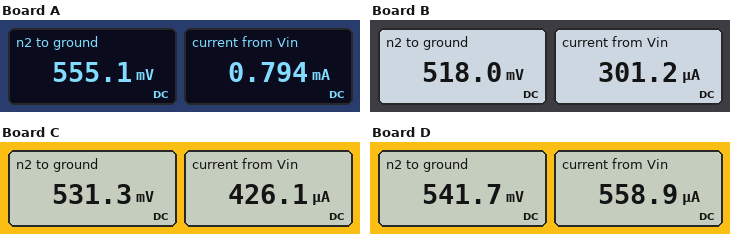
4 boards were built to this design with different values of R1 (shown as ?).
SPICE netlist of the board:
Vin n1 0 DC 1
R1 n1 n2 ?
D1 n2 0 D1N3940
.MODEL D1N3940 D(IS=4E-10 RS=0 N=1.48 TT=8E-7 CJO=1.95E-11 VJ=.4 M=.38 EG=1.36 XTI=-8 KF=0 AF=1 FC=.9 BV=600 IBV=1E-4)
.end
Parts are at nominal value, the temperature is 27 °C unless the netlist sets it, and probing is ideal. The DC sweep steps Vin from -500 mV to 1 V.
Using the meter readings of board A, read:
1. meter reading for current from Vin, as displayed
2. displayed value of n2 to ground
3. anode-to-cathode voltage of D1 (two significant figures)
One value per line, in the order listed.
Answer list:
0.794 mA
555.1 mV
560 mV
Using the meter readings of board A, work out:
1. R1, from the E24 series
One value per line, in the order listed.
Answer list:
560 Ω
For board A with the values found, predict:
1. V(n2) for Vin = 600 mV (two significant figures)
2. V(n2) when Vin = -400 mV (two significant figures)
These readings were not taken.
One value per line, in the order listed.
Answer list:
500 mV
-400 mV
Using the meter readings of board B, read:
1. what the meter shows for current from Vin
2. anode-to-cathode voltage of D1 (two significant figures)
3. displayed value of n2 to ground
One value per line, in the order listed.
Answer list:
301.2 µA
520 mV
518.0 mV
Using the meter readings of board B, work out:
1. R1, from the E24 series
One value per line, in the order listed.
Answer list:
1.6 kΩ
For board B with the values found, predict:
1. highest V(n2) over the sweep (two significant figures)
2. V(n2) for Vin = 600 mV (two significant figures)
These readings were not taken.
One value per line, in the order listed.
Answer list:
520 mV
470 mV
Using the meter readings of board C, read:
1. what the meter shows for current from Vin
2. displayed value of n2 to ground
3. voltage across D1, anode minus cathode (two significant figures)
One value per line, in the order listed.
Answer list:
426.1 µA
531.3 mV
530 mV
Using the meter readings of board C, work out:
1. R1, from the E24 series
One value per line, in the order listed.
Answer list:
1.1 kΩ
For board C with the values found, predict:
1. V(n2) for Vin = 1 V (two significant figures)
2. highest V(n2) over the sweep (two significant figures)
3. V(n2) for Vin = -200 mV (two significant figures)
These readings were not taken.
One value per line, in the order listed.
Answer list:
530 mV
530 mV
-200 mV
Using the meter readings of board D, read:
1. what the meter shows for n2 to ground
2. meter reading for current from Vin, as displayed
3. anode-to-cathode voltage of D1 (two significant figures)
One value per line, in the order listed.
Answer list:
541.7 mV
558.9 µA
540 mV
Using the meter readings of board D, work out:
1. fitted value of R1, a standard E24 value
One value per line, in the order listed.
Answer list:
820 Ω
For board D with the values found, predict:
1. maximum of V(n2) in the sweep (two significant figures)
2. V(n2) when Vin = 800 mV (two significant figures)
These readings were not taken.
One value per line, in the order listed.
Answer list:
540 mV
520 mV
